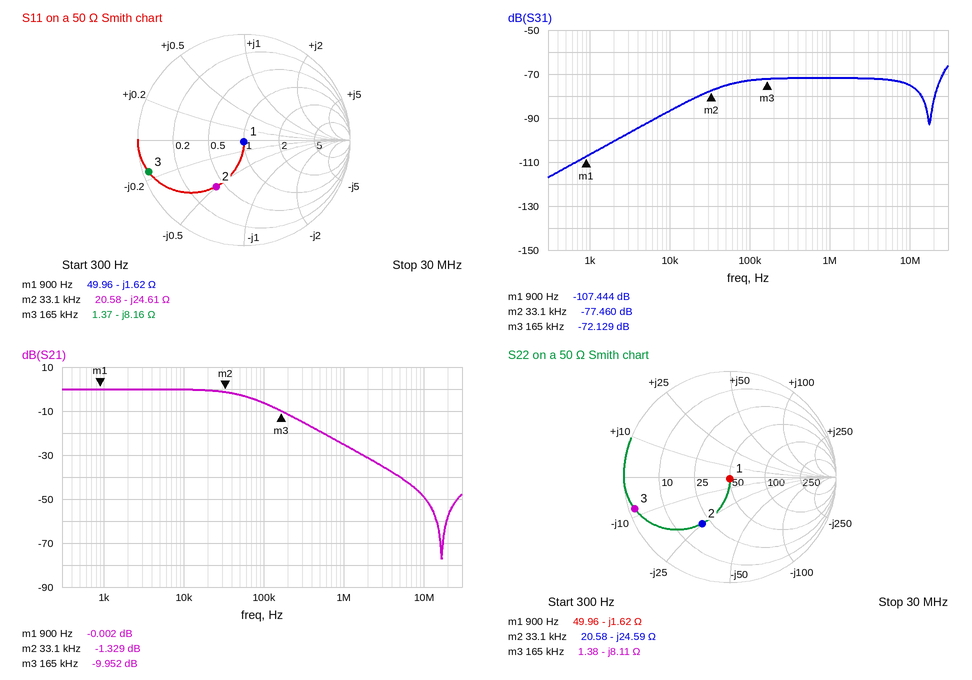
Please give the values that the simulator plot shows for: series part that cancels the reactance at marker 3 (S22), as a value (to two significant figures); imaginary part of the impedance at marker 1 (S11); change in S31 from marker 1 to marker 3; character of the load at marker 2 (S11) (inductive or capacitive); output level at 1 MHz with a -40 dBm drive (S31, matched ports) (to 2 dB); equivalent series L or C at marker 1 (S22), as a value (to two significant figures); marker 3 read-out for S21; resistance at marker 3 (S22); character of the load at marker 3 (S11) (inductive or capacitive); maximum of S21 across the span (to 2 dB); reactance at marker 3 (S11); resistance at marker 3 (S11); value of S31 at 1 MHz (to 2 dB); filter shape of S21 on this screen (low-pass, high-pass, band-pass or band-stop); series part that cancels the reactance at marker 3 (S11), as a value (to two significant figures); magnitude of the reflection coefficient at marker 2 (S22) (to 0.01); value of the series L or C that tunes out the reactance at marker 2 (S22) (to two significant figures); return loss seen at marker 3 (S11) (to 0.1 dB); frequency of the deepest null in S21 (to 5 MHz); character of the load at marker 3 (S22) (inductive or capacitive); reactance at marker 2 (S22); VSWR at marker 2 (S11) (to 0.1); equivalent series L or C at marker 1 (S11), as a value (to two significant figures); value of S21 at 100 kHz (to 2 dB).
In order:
7.8 µH
-1.62 Ω
35.315 dB
capacitive
-112 dBm
110 µF
-9.952 dB
1.38 Ω
capacitive
0 dB
-8.16 Ω
1.37 Ω
-72 dB
low-pass
7.9 µH
0.51
120 µH
0.5 dB
15 MHz
capacitive
-24.59 Ω
3.1
110 µF
-6 dB
